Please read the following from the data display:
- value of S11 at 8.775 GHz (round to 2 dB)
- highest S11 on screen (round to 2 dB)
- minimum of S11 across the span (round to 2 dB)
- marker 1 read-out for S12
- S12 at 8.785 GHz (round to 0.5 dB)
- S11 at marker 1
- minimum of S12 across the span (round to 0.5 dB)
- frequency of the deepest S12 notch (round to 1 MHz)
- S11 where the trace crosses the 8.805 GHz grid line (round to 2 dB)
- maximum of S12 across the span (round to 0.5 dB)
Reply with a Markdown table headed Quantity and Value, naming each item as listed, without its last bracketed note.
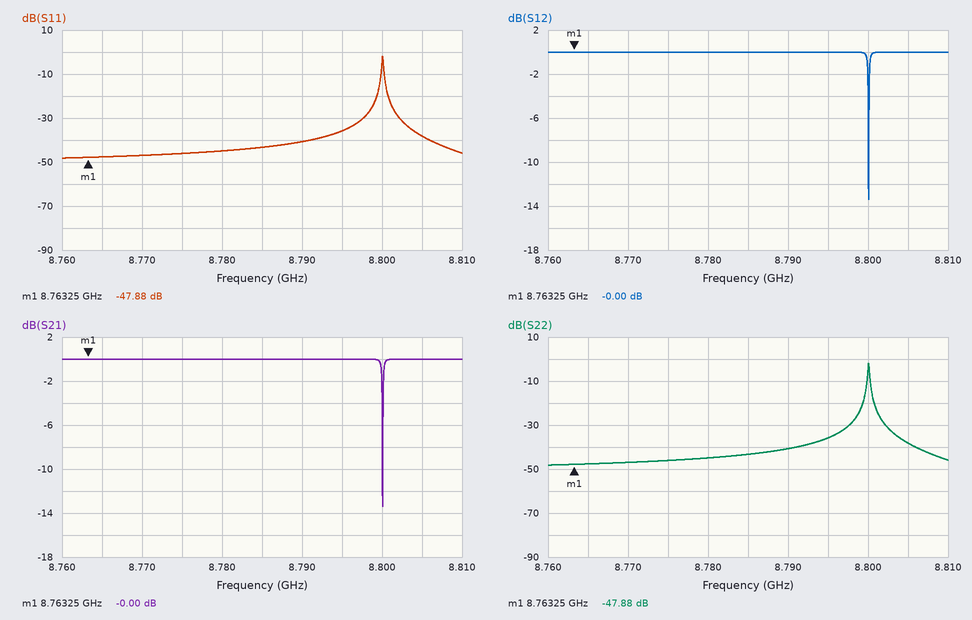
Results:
| Quantity | Value |
|---|---|
| value of S11 at 8.775 GHz | -46 dB |
| highest S11 on screen | -2 dB |
| minimum of S11 across the span | -48 dB |
| marker 1 read-out for S12 | -0.00 dB |
| S12 at 8.785 GHz | 0.0 dB |
| S11 at marker 1 | -47.88 dB |
| minimum of S12 across the span | -13.5 dB |
| frequency of the deepest S12 notch | 8.800 GHz |
| S11 where the trace crosses the 8.805 GHz grid line | -38 dB |
| maximum of S12 across the span | 0.0 dB |
